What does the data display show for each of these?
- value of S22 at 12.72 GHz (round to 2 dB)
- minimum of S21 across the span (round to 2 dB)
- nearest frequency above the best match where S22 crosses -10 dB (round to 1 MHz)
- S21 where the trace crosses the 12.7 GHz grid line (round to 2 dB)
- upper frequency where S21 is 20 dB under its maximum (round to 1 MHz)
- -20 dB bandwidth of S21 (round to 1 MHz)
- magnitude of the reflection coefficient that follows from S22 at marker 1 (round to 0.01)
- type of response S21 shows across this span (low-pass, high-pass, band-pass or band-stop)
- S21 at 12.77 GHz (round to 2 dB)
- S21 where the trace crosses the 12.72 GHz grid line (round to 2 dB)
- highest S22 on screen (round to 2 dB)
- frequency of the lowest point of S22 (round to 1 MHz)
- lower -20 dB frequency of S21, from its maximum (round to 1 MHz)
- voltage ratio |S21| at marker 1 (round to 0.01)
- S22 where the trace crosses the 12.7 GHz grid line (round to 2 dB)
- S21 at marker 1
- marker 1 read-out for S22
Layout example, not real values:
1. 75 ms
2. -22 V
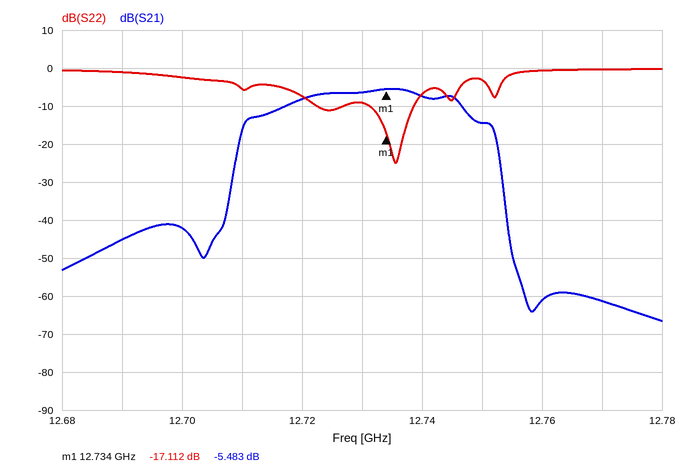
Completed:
1. -8 dB
2. -66 dB
3. 12.739 GHz
4. -42 dB
5. 12.753 GHz
6. 44 MHz
7. 0.14
8. band-pass
9. -62 dB
10. -8 dB
11. 0 dB
12. 12.736 GHz
13. 12.709 GHz
14. 0.53
15. -2 dB
16. -5.483 dB
17. -17.112 dB
